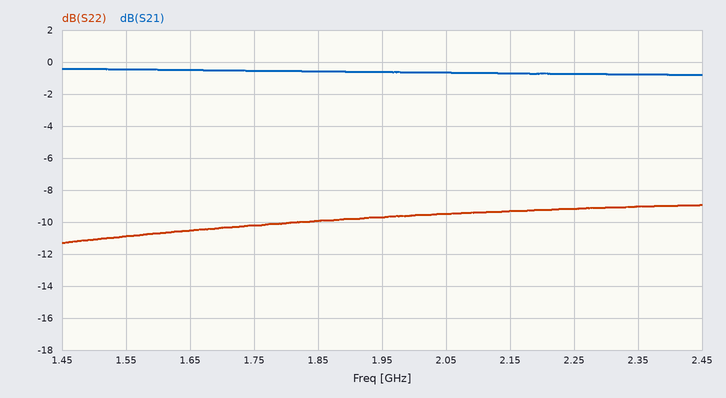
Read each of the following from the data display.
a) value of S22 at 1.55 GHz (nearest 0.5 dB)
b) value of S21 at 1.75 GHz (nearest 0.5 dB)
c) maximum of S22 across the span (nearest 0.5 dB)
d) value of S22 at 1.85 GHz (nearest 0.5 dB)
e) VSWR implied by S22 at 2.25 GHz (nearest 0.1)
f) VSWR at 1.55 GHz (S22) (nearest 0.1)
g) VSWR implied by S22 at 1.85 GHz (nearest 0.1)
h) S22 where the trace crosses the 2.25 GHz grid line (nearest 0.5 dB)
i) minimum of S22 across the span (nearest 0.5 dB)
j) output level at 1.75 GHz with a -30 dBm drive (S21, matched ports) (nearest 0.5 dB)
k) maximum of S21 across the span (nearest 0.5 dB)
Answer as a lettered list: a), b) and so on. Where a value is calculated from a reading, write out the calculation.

a) -11.0 dB
b) -0.5 dB
c) -9.0 dB
d) -10.0 dB
e) |Γ| = 10^(-9/20) = 0.3548; VSWR = (1 + 0.3548)/(1 − 0.3548) ≈ 2.1
f) |Γ| = 10^(-11/20) = 0.2818; VSWR = (1 + 0.2818)/(1 − 0.2818) ≈ 1.8
g) |Γ| = 10^(-10/20) = 0.3162; VSWR = (1 + 0.3162)/(1 − 0.3162) ≈ 1.9
h) -9.0 dB
i) -11.5 dB
j) -30 dBm + (-0.5 dB) = -30.5 dBm
k) -0.5 dB
